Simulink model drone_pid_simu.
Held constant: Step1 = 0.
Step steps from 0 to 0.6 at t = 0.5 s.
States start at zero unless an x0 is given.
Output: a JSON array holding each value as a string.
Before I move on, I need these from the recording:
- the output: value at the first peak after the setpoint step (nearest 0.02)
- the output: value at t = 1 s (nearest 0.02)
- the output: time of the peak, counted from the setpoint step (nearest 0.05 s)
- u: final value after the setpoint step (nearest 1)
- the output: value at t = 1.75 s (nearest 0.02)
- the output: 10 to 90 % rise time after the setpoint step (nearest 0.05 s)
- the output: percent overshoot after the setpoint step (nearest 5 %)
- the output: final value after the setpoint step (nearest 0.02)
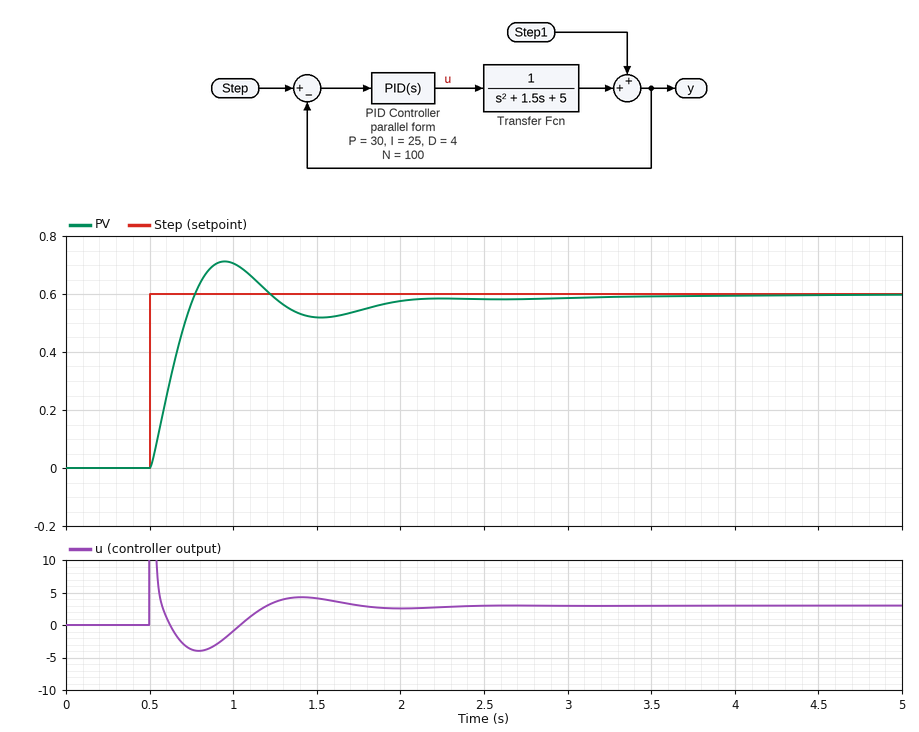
["0.72", "0.70", "0.45 s", "3", "0.54", "0.20 s", "20 %", "0.60"]
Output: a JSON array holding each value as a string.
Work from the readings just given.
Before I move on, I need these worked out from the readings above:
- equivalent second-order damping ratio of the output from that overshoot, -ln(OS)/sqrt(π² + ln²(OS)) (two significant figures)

["0.46"]
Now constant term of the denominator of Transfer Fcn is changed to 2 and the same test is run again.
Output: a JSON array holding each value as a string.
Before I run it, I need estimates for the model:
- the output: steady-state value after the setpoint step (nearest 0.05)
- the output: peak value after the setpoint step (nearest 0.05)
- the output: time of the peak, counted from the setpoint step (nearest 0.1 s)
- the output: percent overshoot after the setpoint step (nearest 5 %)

["0.60", "0.75", "0.5 s", "25 %"]
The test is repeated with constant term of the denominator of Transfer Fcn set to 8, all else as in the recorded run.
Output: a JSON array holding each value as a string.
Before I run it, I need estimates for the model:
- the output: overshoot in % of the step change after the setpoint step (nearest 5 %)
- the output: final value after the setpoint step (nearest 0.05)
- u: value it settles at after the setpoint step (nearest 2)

["10 %", "0.60", "4"]
